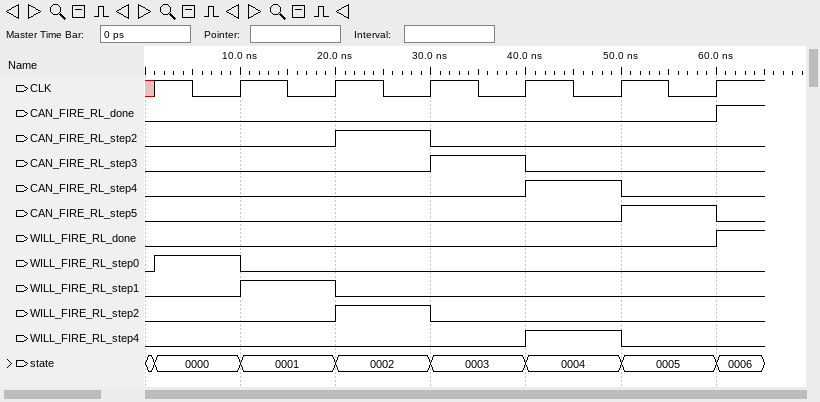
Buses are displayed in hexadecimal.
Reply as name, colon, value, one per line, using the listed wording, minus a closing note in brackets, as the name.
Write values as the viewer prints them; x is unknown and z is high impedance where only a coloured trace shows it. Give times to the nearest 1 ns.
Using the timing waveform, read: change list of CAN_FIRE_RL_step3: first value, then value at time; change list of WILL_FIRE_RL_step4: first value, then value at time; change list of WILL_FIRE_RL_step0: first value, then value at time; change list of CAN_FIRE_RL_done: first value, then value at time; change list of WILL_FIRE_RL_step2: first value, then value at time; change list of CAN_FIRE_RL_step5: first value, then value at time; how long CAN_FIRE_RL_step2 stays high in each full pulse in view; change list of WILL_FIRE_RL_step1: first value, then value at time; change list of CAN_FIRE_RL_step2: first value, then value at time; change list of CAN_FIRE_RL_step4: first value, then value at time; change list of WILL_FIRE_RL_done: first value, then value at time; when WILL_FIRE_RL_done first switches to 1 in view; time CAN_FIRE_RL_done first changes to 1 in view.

change list of CAN_FIRE_RL_step3: first value, then value at time: 0, 1 at 30 ns, 0 at 40 ns
change list of WILL_FIRE_RL_step4: first value, then value at time: 0, 1 at 40 ns, 0 at 50 ns
change list of WILL_FIRE_RL_step0: first value, then value at time: 0, 1 at 1 ns, 0 at 10 ns
change list of CAN_FIRE_RL_done: first value, then value at time: 0, 1 at 60 ns
change list of WILL_FIRE_RL_step2: first value, then value at time: 0, 1 at 20 ns, 0 at 30 ns
change list of CAN_FIRE_RL_step5: first value, then value at time: 0, 1 at 50 ns, 0 at 60 ns
how long CAN_FIRE_RL_step2 stays high in each full pulse in view: 10 ns
change list of WILL_FIRE_RL_step1: first value, then value at time: 0, 1 at 10 ns, 0 at 20 ns
change list of CAN_FIRE_RL_step2: first value, then value at time: 0, 1 at 20 ns, 0 at 30 ns
change list of CAN_FIRE_RL_step4: first value, then value at time: 0, 1 at 40 ns, 0 at 50 ns
change list of WILL_FIRE_RL_done: first value, then value at time: 0, 1 at 60 ns
when WILL_FIRE_RL_done first switches to 1 in view: 60 ns
time CAN_FIRE_RL_done first changes to 1 in view: 60 ns
